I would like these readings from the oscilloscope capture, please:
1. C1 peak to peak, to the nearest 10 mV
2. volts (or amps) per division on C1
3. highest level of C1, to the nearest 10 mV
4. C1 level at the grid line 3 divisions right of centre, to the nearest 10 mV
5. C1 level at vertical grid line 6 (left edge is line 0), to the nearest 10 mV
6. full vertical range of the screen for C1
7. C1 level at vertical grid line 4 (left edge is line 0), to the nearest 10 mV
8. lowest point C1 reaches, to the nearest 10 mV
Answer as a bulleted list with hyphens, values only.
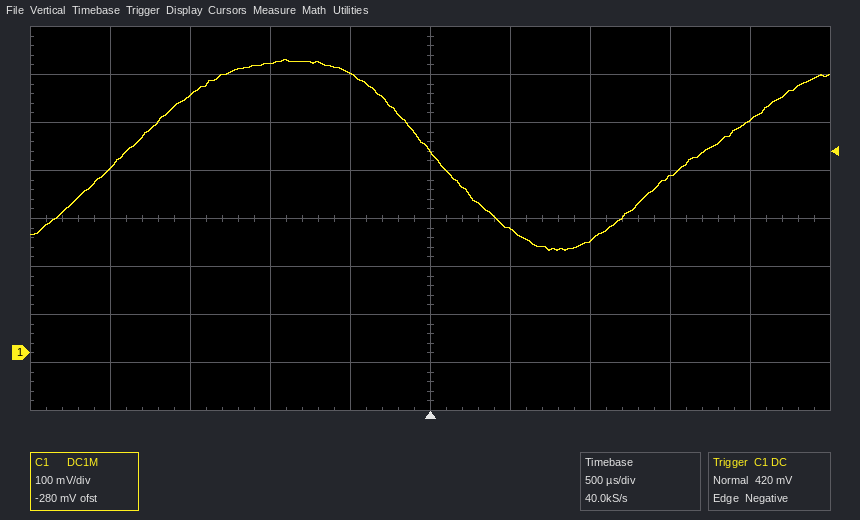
- 400 mV
- 100 mV
- 610 mV
- 370 mV
- 260 mV
- 800 mV
- 580 mV
- 210 mV
